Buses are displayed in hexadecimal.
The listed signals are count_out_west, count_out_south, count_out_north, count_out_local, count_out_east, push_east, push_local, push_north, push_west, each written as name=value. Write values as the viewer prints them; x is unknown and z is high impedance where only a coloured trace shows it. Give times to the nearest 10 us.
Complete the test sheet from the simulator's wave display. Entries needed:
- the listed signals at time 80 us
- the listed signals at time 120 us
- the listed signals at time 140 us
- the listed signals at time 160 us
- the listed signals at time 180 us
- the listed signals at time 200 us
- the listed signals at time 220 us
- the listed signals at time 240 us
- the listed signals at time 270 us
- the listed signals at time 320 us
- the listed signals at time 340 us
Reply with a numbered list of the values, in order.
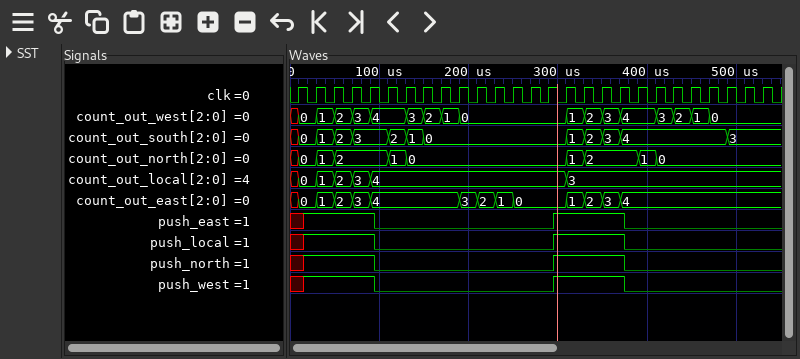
1. count_out_west=3, count_out_south=3, count_out_north=2, count_out_local=3, count_out_east=3, push_east=1, push_local=1, push_north=1, push_west=1
2. count_out_west=4, count_out_south=2, count_out_north=1, count_out_local=4, count_out_east=4, push_east=0, push_local=0, push_north=0, push_west=0
3. count_out_west=3, count_out_south=1, count_out_north=0, count_out_local=4, count_out_east=4, push_east=0, push_local=0, push_north=0, push_west=0
4. count_out_west=2, count_out_south=0, count_out_north=0, count_out_local=4, count_out_east=4, push_east=0, push_local=0, push_north=0, push_west=0
5. count_out_west=1, count_out_south=0, count_out_north=0, count_out_local=4, count_out_east=4, push_east=0, push_local=0, push_north=0, push_west=0
6. count_out_west=0, count_out_south=0, count_out_north=0, count_out_local=4, count_out_east=3, push_east=0, push_local=0, push_north=0, push_west=0
7. count_out_west=0, count_out_south=0, count_out_north=0, count_out_local=4, count_out_east=2, push_east=0, push_local=0, push_north=0, push_west=0
8. count_out_west=0, count_out_south=0, count_out_north=0, count_out_local=4, count_out_east=1, push_east=0, push_local=0, push_north=0, push_west=0
9. count_out_west=0, count_out_south=0, count_out_north=0, count_out_local=4, count_out_east=0, push_east=0, push_local=0, push_north=0, push_west=0
10. count_out_west=1, count_out_south=1, count_out_north=1, count_out_local=3, count_out_east=1, push_east=1, push_local=1, push_north=1, push_west=1
11. count_out_west=2, count_out_south=2, count_out_north=2, count_out_local=3, count_out_east=2, push_east=1, push_local=1, push_north=1, push_west=1
